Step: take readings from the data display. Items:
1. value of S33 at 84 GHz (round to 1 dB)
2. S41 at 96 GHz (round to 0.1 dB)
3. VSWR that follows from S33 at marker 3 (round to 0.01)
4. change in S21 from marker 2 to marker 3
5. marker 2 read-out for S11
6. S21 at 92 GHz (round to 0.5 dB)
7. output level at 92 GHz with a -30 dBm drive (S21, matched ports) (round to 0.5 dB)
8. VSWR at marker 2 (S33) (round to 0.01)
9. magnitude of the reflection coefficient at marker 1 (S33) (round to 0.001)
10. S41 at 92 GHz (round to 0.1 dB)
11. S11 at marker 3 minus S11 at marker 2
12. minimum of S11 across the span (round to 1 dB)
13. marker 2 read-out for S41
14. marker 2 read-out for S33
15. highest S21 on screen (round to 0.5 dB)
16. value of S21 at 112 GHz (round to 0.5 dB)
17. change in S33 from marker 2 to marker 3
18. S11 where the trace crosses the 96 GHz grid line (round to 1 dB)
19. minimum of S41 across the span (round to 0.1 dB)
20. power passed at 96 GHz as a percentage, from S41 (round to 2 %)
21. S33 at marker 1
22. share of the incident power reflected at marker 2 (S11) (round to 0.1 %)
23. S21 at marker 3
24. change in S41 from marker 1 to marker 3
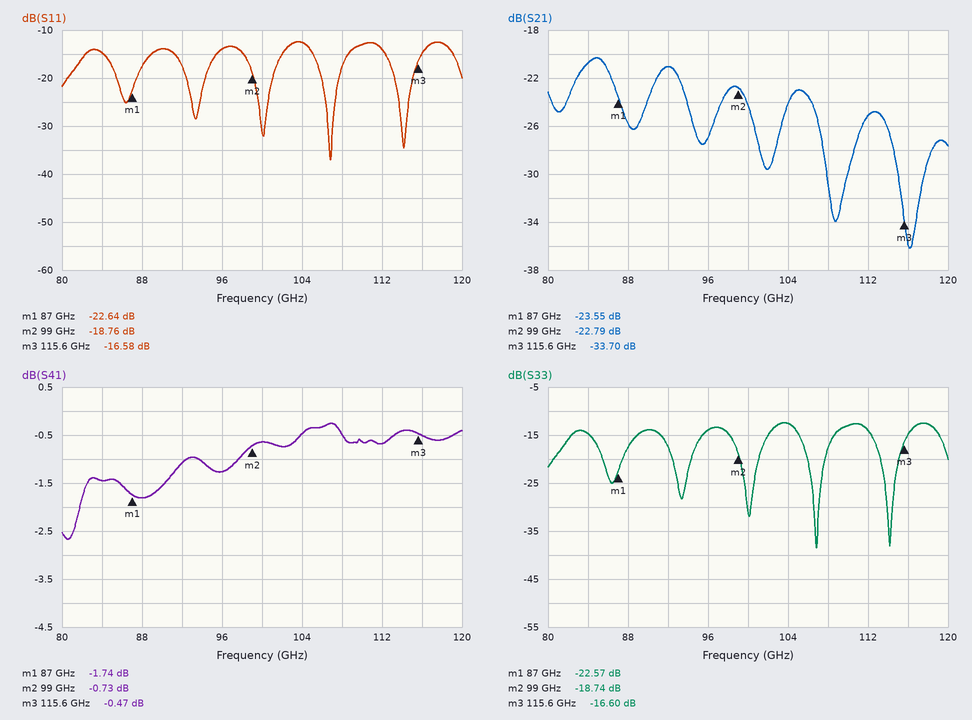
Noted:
-15 dB
-1.3 dB
1.35
-10.91 dB
-18.76 dB
-21.0 dB
-51.0 dBm
1.26
0.074
-1.1 dB
2.18 dB
-37 dB
-0.73 dB
-18.74 dB
-20.5 dB
-25.0 dB
2.14 dB
-14 dB
-2.7 dB
74 %
-22.57 dB
1.3 %
-33.70 dB
1.27 dB
